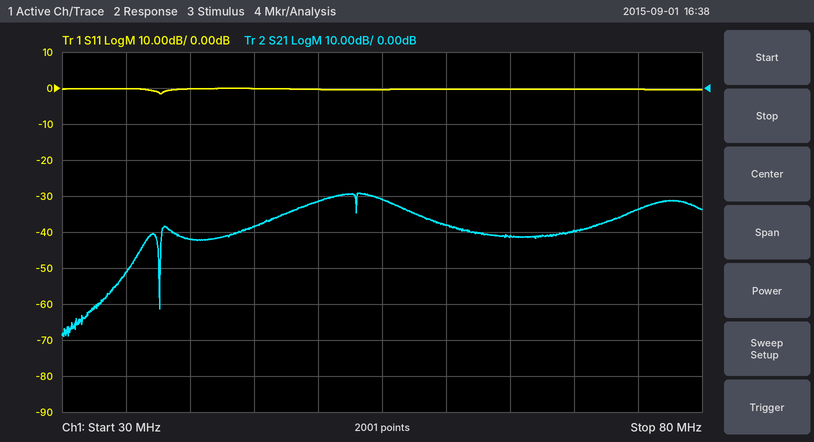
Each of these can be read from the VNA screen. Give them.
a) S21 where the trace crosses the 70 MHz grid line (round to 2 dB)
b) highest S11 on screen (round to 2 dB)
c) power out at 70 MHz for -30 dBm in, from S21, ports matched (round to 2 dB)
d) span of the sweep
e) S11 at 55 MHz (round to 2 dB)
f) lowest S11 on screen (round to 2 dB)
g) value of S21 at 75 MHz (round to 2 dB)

-40 dB
0 dB
-70 dBm
50 MHz
0 dB
-2 dB
-34 dB
